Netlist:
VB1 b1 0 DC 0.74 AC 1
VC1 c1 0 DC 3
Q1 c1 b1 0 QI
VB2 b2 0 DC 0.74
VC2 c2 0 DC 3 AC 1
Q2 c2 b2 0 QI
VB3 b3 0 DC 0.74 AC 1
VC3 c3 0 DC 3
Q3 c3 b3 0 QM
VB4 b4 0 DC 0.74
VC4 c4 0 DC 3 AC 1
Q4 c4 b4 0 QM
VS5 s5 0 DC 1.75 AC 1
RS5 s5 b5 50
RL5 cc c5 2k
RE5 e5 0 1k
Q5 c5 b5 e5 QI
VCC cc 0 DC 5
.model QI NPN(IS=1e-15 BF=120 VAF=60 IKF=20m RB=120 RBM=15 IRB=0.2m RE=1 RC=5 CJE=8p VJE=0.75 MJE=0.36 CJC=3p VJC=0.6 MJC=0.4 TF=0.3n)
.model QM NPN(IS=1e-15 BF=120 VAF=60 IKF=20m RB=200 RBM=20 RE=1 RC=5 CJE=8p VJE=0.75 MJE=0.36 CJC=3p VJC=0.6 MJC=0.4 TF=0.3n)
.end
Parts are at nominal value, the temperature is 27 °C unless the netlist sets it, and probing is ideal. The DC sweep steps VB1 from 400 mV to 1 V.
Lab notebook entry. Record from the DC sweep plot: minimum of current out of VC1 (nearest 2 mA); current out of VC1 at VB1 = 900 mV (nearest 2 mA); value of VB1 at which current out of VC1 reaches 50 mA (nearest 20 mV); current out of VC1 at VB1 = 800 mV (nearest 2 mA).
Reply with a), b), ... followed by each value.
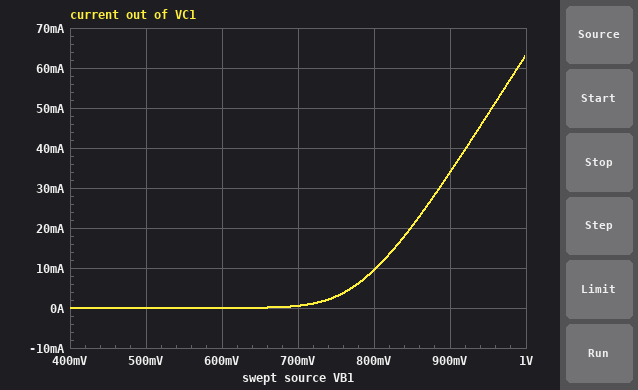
a) 0 A
b) 34 mA
c) 960 mV
d) 10 mA
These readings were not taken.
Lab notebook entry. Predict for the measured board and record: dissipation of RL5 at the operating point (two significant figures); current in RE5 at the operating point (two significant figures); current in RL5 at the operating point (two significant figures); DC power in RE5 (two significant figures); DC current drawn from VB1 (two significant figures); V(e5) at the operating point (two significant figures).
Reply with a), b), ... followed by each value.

a) 2.1 mW
b) 1.0 mA
c) 1.0 mA
d) 1.1 mW
e) 19 µA
f) 1.0 V
